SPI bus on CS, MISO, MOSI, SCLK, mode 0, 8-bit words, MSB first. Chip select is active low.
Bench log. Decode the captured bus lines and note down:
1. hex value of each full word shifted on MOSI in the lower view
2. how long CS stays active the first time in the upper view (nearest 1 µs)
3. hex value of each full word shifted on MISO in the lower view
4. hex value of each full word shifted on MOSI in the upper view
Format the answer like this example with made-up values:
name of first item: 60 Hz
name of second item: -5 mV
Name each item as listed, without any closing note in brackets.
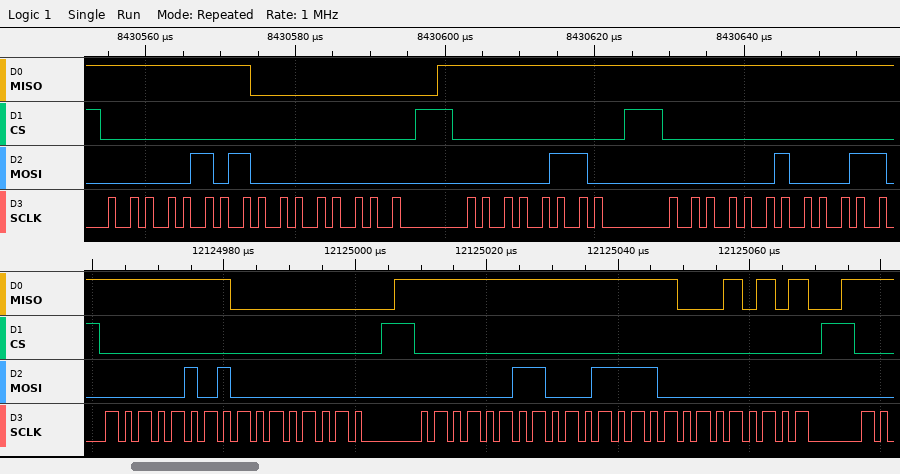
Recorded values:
hex value of each full word shifted on MOSI in the lower view: 05, 00, 03, 1E, 00
how long CS stays active the first time in the upper view: 42 µs
hex value of each full word shifted on MISO in the lower view: FF, 00, FF, FF, 15
hex value of each full word shifted on MOSI in the upper view: 05, 00, 06, 02
